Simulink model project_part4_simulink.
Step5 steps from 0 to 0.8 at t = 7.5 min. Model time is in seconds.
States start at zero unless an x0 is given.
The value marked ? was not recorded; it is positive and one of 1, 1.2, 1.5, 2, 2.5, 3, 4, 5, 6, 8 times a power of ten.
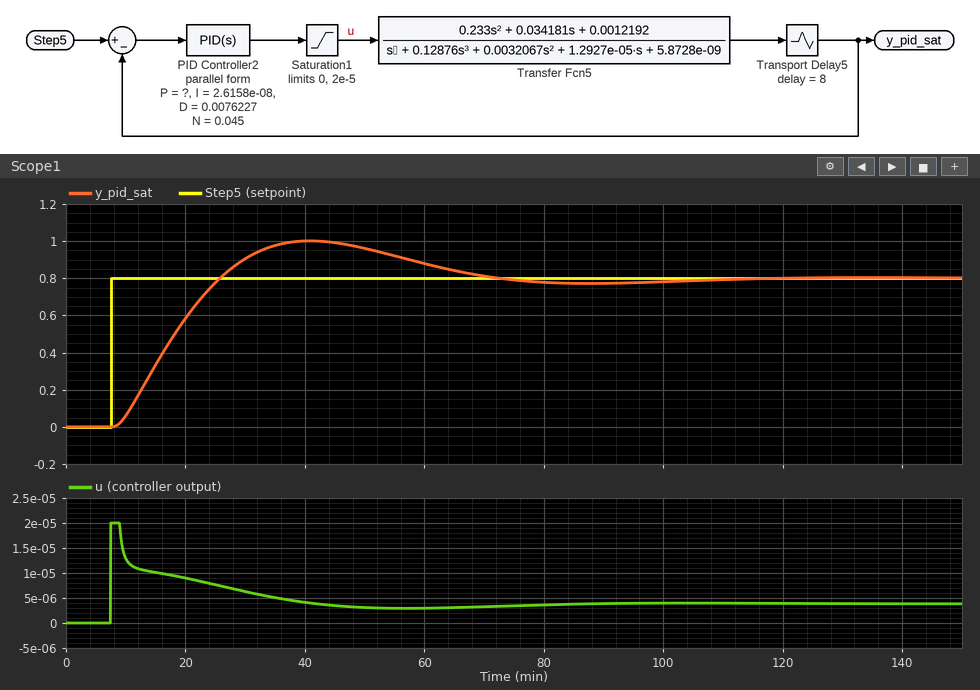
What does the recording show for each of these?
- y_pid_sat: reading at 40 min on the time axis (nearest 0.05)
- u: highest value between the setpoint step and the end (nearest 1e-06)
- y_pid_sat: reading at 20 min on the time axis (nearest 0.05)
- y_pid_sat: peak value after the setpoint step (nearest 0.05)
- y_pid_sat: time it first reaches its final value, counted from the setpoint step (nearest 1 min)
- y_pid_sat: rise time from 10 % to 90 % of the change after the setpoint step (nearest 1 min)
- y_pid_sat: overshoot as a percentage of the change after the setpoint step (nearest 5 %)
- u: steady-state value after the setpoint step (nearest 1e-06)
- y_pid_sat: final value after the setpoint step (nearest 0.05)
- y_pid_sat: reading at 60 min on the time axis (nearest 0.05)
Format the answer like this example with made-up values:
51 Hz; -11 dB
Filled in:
1.00; 0.000020; 0.60; 1.00; 18 min; 13 min; 25 %; 0.000004; 0.80; 0.90
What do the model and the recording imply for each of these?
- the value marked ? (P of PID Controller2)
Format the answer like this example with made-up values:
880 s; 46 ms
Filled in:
2e-05
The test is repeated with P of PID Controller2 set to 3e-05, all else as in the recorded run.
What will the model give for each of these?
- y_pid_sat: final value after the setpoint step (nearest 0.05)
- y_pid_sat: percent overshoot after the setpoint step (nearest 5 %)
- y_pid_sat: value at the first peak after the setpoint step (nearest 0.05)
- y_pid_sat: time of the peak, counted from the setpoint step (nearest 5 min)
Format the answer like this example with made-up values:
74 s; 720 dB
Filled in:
0.80; 15 %; 0.95; 30 min
